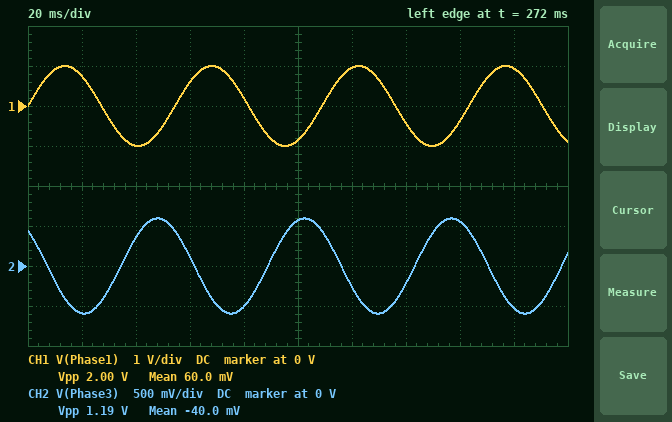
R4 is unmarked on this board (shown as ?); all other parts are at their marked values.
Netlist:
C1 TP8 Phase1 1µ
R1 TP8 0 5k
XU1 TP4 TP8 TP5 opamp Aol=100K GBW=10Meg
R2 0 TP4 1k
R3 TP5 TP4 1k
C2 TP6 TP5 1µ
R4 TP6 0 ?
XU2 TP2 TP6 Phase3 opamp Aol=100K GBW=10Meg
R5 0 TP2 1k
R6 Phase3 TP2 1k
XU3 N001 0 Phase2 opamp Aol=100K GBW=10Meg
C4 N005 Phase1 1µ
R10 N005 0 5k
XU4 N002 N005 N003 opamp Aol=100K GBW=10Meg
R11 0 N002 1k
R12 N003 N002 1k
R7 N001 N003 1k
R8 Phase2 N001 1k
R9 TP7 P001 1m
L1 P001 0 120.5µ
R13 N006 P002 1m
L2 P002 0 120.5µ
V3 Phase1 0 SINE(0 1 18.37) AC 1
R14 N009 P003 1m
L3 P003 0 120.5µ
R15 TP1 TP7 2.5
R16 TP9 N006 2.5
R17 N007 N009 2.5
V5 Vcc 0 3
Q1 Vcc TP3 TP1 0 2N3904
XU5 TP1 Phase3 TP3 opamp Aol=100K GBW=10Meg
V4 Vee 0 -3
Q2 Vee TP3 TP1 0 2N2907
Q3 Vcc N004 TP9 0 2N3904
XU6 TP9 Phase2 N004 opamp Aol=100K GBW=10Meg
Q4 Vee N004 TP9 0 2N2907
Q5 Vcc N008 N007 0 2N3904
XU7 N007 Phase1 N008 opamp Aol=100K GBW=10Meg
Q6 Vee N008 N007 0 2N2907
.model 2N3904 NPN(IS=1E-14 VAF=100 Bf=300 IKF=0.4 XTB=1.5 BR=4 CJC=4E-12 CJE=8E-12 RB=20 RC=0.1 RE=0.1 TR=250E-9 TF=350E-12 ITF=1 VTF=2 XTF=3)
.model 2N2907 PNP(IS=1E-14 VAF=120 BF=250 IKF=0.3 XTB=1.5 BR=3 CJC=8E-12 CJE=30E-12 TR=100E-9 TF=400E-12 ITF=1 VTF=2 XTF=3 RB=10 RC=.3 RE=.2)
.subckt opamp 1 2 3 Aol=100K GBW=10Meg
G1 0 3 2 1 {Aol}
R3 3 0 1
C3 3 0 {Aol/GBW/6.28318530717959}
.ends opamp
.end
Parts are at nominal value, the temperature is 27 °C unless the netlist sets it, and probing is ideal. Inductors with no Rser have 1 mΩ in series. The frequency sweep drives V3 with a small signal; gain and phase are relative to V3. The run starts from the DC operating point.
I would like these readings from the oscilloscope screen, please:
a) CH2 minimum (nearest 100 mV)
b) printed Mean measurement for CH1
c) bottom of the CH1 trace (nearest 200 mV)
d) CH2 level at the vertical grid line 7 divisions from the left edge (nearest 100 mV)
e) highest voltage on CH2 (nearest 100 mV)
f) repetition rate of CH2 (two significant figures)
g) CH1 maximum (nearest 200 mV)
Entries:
-600 mV
60.0 mV
-1.0 V
-200 mV
600 mV
18 Hz
1.0 V
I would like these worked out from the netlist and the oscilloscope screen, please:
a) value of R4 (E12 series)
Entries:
2.7 kΩ
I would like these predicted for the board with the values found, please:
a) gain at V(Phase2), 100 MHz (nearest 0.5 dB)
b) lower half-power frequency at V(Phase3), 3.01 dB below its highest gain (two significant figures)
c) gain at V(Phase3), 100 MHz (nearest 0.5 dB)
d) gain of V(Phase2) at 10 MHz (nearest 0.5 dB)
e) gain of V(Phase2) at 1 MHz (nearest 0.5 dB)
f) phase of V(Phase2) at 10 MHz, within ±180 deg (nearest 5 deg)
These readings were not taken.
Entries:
-46.0 dB
72 Hz
-40.0 dB
-8.0 dB
5.5 dB
55 deg
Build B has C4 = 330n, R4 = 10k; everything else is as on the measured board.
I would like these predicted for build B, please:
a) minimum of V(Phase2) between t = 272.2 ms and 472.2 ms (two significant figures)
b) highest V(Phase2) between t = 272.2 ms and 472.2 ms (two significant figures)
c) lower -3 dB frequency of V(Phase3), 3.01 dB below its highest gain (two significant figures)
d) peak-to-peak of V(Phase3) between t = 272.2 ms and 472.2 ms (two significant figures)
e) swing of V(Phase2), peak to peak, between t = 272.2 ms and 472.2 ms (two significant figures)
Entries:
-370 mV
370 mV
38 Hz
3.0 V
750 mV
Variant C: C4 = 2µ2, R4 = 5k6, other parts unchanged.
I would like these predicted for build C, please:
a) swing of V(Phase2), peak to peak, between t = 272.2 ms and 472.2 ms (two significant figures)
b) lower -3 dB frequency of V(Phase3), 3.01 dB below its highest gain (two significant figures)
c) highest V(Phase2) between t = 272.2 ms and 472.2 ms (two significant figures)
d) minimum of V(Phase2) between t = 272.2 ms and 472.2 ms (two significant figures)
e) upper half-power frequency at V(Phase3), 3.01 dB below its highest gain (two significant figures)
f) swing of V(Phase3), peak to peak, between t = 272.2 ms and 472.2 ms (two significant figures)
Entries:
3.1 V
47 Hz
1.6 V
-1.6 V
3.2 MHz
2.2 V
